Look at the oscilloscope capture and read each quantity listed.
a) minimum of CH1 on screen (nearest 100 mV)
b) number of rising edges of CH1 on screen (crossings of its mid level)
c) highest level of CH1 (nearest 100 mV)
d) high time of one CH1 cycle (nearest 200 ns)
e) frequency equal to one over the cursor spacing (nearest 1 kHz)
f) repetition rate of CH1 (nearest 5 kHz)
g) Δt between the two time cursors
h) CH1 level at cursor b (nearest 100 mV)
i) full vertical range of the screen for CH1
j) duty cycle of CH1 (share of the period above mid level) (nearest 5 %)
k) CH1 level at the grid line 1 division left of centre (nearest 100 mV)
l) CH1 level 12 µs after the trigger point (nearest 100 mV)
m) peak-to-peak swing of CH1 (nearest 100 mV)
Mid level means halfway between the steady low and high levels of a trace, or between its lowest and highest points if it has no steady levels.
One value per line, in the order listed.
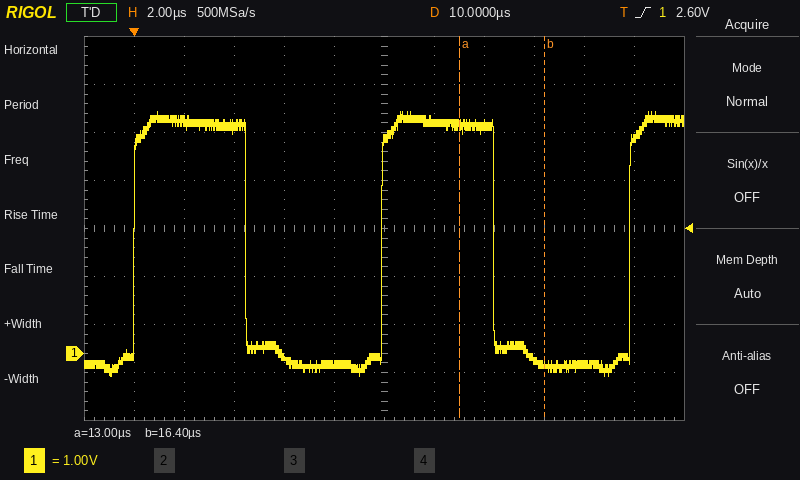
-500 mV
3
5.0 V
4.4 µs
294 kHz
100 kHz
3.4 µs
-200 mV
8 V
45 %
-200 mV
4.8 V
5.5 V
